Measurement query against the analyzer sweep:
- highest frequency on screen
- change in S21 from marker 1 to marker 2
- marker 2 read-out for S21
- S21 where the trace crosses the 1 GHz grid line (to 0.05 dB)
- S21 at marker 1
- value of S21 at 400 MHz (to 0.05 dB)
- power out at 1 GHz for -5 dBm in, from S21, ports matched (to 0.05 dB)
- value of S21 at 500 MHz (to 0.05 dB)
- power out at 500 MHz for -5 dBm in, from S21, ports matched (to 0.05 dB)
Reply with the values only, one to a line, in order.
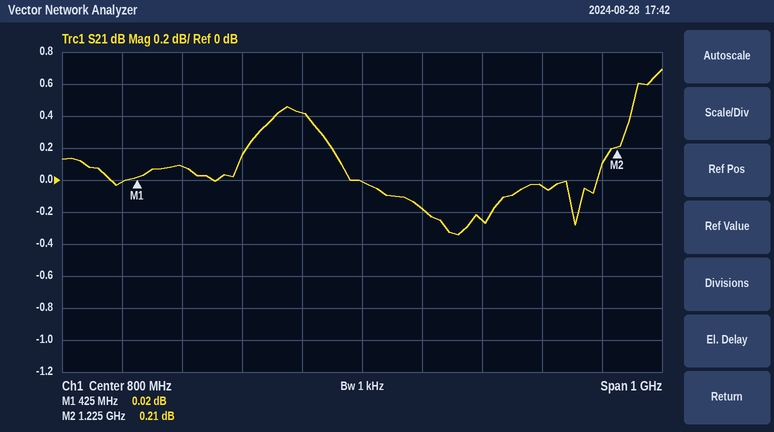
1.3 GHz
0.19 dB
0.21 dB
-0.25 dB
0.02 dB
0.00 dB
-5.25 dBm
0.10 dB
-4.90 dBm
